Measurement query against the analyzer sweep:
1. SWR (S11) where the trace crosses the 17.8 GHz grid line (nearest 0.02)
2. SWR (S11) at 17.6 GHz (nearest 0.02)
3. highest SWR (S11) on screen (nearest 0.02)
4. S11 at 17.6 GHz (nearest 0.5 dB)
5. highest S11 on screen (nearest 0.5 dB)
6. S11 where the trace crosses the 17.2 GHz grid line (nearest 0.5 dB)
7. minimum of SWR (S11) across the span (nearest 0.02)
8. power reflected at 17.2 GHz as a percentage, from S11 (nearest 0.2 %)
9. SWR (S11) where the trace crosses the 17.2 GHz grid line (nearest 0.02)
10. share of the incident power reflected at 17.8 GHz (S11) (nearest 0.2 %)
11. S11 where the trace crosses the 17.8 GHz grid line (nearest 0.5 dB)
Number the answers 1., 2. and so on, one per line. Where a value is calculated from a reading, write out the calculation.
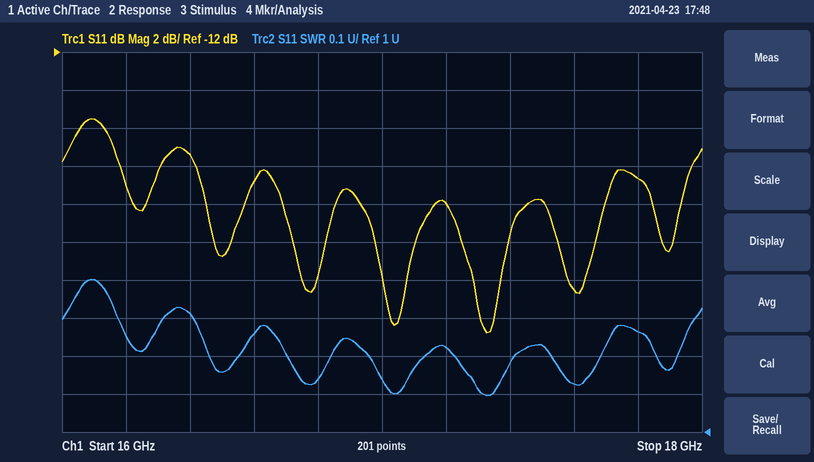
1. 1.26
2. 1.12
3. 1.40
4. -24.5 dB
5. -15.5 dB
6. -20.0 dB
7. 1.10
8. 10^(-20/10) ≈ 1.0 %
9. 1.22
10. 10^(-18.5/10) ≈ 1.4 %
11. -18.5 dB
